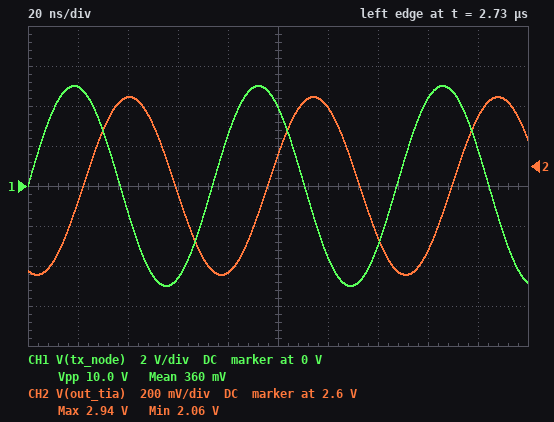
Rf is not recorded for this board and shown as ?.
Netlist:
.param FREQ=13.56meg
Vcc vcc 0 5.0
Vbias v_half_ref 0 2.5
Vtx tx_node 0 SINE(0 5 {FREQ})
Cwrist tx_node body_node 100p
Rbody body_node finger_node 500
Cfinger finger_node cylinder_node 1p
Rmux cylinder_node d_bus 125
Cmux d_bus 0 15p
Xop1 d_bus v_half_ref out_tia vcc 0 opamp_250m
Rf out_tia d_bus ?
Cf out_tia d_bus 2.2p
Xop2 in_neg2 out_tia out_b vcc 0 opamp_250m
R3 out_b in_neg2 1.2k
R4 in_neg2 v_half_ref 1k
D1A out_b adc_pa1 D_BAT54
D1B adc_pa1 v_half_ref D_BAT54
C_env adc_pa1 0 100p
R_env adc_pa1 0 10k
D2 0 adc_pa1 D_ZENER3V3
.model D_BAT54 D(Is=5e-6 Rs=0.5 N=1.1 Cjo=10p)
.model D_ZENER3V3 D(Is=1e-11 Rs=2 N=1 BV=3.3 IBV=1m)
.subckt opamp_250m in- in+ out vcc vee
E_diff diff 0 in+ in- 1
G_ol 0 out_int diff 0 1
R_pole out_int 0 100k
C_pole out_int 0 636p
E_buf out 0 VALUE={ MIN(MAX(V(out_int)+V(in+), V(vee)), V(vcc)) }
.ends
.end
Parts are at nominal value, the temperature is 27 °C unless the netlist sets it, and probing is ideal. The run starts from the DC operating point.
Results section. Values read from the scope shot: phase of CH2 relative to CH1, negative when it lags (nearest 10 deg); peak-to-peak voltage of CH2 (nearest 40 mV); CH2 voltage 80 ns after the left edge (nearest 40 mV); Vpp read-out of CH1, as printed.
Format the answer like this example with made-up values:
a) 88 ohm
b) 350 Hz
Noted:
a) -110 deg
b) 880 mV
c) 2.08 V
d) 10.0 V
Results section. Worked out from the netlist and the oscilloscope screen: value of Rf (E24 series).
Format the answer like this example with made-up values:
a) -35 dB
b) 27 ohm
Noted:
a) 1 kΩ
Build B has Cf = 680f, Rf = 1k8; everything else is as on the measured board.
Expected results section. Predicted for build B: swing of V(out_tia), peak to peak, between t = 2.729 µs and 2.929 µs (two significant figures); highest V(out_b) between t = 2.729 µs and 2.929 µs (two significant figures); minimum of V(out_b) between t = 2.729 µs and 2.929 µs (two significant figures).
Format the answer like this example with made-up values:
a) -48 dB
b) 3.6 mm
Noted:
a) 1.7 V
b) 4.4 V
c) 610 mV
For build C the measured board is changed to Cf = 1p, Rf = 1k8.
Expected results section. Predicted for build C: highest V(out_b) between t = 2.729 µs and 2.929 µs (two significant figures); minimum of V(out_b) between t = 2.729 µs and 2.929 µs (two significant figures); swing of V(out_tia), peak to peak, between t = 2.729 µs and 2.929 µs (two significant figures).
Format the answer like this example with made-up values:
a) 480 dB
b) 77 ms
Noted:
a) 4.4 V
b) 620 mV
c) 1.7 V
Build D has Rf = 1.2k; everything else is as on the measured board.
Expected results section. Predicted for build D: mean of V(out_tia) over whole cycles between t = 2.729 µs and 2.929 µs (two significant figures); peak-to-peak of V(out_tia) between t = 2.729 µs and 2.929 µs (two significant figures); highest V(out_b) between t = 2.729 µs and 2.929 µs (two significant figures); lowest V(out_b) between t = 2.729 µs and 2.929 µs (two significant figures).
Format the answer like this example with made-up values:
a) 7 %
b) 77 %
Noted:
a) 2.5 V
b) 1.1 V
c) 3.7 V
d) 1.3 V
